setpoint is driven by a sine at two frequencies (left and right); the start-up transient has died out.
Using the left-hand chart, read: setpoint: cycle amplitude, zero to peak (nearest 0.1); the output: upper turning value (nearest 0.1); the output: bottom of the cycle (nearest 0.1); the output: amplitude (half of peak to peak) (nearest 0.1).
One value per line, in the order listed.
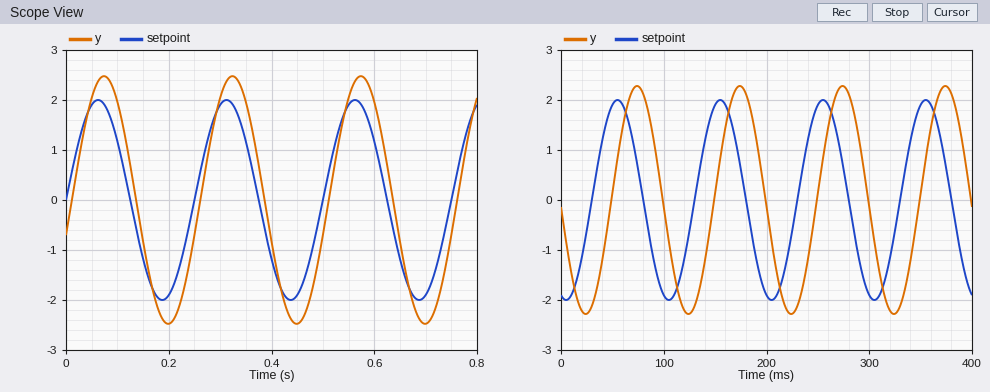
2.0
2.5
-2.5
2.5
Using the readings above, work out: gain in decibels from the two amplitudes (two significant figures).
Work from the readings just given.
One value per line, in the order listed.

1.9 dB
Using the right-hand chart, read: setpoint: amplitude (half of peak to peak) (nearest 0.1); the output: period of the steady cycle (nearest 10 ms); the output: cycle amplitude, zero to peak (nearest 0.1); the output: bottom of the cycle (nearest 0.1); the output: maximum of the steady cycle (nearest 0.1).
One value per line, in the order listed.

2.0
100 ms
2.3
-2.3
2.3
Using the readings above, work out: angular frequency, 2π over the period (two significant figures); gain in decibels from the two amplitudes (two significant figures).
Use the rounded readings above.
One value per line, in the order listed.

0.063 rad/ms
1.2 dB
